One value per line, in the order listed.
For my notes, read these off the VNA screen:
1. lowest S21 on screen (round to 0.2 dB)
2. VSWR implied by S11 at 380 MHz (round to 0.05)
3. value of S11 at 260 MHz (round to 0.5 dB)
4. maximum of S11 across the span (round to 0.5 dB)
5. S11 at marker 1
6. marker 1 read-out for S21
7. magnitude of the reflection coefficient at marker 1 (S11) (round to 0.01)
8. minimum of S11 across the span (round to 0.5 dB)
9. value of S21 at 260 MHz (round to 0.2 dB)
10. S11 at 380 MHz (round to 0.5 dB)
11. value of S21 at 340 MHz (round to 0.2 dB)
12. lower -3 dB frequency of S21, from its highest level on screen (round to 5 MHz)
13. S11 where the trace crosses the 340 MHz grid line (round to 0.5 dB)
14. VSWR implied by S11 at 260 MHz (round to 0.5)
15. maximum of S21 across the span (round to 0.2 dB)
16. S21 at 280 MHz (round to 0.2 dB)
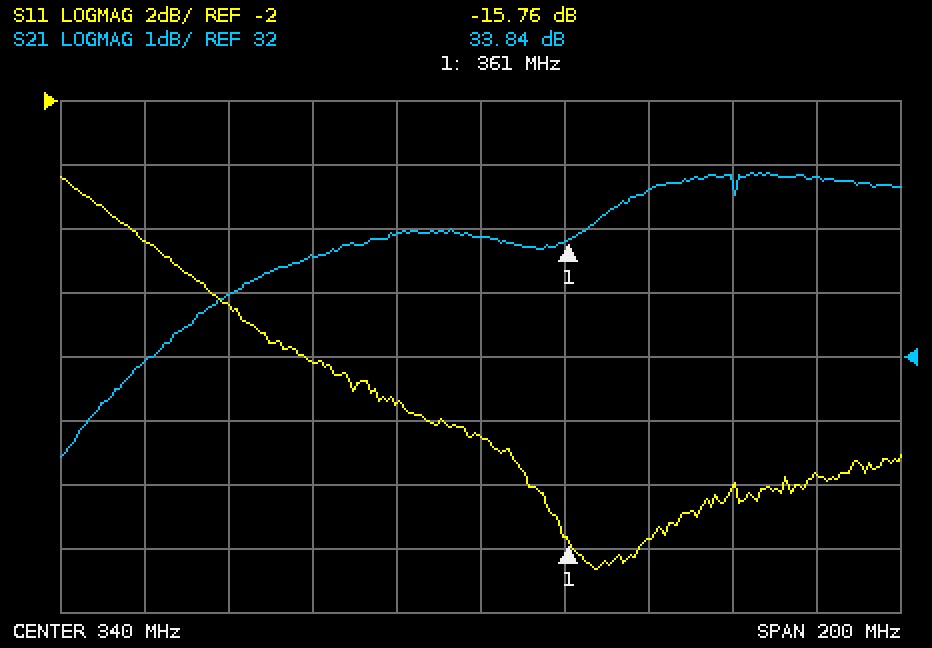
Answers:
30.4 dB
1.40
-6.5 dB
-4.5 dB
-15.76 dB
33.84 dB
0.16
-16.5 dB
32.0 dB
-15.5 dB
33.8 dB
260 MHz
-12.5 dB
3.0
34.8 dB
33.0 dB
